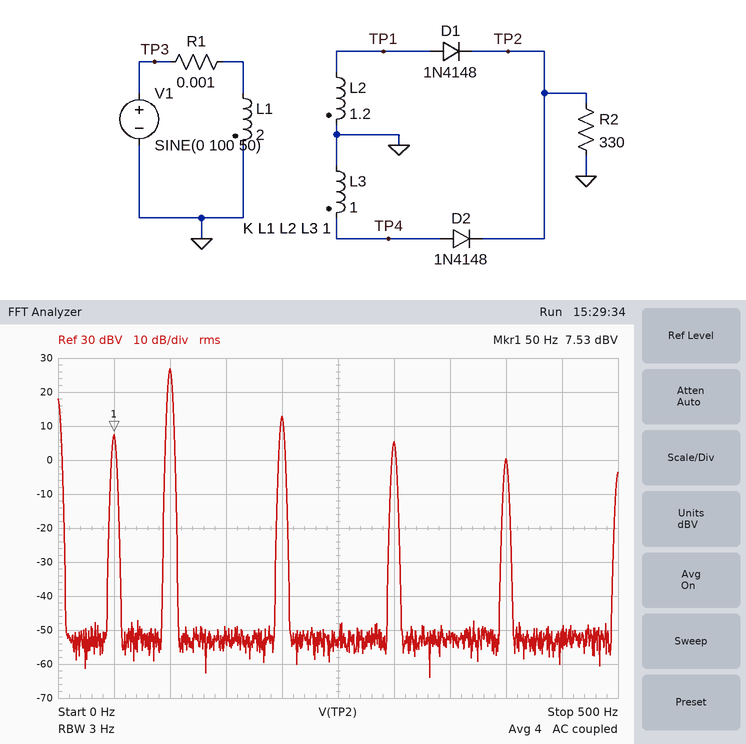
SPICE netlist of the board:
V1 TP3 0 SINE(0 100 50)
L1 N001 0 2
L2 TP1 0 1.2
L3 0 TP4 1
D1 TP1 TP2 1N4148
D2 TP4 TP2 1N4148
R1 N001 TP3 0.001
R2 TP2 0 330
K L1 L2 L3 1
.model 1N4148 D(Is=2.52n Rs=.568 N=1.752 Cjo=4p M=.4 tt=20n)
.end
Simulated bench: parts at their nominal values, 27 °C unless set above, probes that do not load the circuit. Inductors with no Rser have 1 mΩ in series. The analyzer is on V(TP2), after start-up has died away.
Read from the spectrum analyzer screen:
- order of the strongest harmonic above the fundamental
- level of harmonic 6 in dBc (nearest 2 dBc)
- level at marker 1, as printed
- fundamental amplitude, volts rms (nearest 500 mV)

2
-2 dBc
7.53 dBV
2.5 V
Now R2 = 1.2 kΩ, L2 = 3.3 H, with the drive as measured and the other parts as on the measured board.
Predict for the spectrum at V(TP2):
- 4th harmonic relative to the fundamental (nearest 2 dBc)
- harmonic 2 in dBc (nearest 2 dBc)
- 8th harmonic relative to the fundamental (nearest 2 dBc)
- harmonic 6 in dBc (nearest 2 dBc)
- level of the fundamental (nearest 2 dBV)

-10 dBc
4 dBc
-24 dBc
-18 dBc
26 dBV
